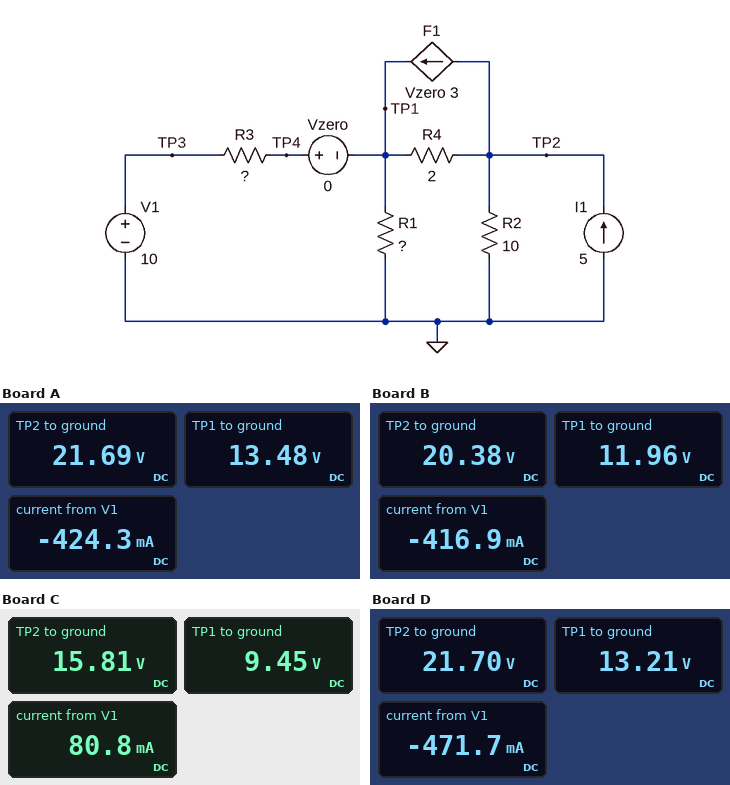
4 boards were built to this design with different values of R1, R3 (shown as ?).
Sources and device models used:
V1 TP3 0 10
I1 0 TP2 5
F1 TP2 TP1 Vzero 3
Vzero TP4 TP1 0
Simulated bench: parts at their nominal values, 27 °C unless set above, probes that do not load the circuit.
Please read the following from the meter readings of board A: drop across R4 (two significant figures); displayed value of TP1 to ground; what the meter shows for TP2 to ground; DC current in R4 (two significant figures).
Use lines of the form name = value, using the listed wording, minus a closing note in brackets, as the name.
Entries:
drop across R4 = 8.2 V
displayed value of TP1 to ground = 13.48 V
what the meter shows for TP2 to ground = 21.69 V
DC current in R4 = 4.1 A
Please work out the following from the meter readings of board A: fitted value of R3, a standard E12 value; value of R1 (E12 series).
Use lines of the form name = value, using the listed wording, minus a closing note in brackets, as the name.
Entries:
fitted value of R3, a standard E12 value = 8.2 Ω
value of R1 = 5.6 Ω
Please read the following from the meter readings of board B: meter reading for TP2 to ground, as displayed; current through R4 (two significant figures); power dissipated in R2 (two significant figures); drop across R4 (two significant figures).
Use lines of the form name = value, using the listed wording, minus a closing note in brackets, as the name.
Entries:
meter reading for TP2 to ground, as displayed = 20.38 V
current through R4 = 4.2 A
power dissipated in R2 = 42 W
drop across R4 = 8.4 V
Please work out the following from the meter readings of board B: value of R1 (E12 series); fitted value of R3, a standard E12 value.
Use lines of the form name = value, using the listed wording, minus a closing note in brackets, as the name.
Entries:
value of R1 = 4.7 Ω
fitted value of R3, a standard E12 value = 4.7 Ω
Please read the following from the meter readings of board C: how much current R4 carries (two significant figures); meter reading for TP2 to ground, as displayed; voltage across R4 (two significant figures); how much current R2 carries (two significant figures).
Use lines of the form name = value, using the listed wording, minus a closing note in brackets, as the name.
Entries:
how much current R4 carries = 3.2 A
meter reading for TP2 to ground, as displayed = 15.81 V
voltage across R4 = 6.4 V
how much current R2 carries = 1.6 A
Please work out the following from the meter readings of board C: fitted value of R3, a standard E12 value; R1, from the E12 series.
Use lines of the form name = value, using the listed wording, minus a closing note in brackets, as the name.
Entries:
fitted value of R3, a standard E12 value = 6.8 Ω
R1, from the E12 series = 2.7 Ω
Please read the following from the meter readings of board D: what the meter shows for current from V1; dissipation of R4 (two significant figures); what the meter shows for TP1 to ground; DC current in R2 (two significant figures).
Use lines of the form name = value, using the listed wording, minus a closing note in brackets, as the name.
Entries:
what the meter shows for current from V1 = -471.7 mA
dissipation of R4 = 36 W
what the meter shows for TP1 to ground = 13.21 V
DC current in R2 = 2.2 A
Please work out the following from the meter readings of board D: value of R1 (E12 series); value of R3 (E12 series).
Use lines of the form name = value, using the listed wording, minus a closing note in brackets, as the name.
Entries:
value of R1 = 5.6 Ω
value of R3 = 6.8 Ω
